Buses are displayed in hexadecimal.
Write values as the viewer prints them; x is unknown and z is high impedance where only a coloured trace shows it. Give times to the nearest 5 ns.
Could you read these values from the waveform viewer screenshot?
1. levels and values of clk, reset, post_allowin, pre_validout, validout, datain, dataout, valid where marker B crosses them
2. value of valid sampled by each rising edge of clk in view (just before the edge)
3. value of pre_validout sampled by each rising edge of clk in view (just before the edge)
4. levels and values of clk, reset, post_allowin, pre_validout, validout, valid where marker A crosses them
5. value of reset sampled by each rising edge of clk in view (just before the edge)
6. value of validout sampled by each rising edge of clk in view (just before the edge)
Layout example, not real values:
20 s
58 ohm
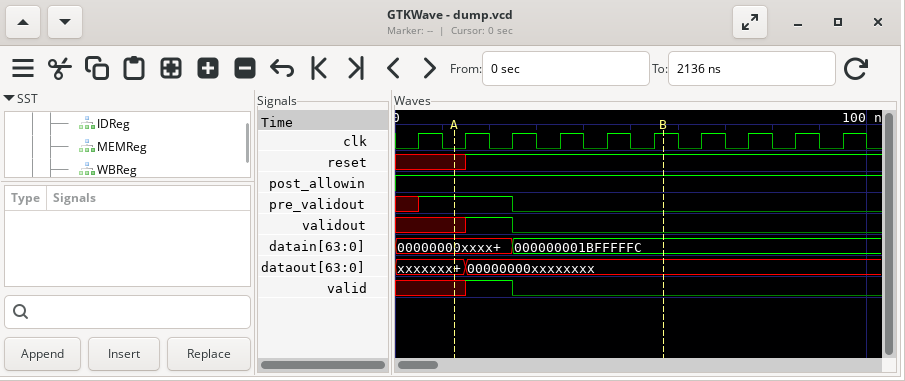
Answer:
clk=1, reset=1, post_allowin=1, pre_validout=0, validout=0, datain=000000001BFFFFFC, dataout=00000000xxxxxxxx, valid=0
x x 1 0 0 0 0 0 0 0
x 1 1 0 0 0 0 0 0 0
clk=0, reset=x, post_allowin=1, pre_validout=1, validout=x, valid=x
x x 1 1 1 1 1 1 1 1
x x 1 0 0 0 0 0 0 0
